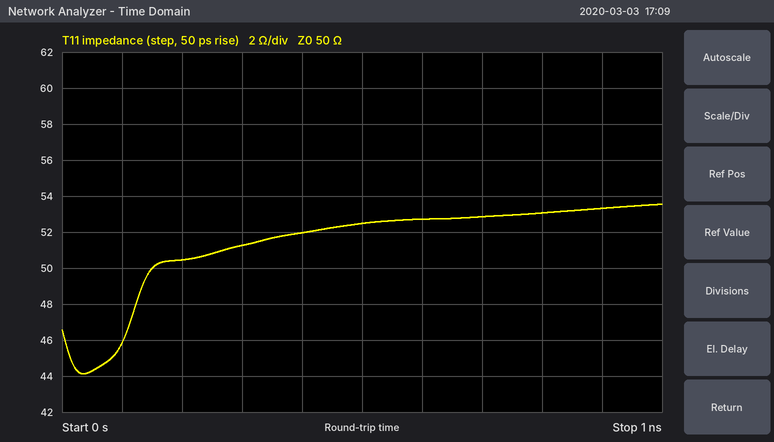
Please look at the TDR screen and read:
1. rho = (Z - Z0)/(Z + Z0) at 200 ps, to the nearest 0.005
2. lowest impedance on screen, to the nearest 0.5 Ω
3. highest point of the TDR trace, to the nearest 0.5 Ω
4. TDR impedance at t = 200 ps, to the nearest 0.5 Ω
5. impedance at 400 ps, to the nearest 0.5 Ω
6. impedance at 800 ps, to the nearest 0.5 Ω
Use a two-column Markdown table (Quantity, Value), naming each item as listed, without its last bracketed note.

| Quantity | Value |
|---|---|
| rho = (Z - Z0)/(Z + Z0) at 200 ps, to the nearest 0.005 | +0.005 |
| lowest impedance on screen, to the nearest 0.5 Ω | 44.0 Ω |
| highest point of the TDR trace, to the nearest 0.5 Ω | 53.5 Ω |
| TDR impedance at t = 200 ps, to the nearest 0.5 Ω | 50.5 Ω |
| impedance at 400 ps, to the nearest 0.5 Ω | 52.0 Ω |
| impedance at 800 ps, to the nearest 0.5 Ω | 53.0 Ω |
